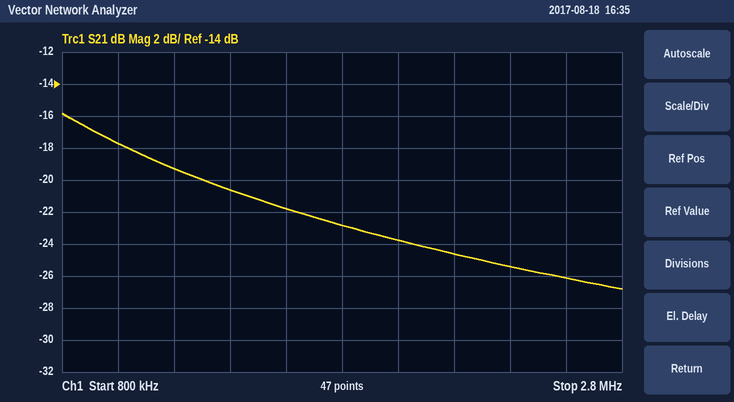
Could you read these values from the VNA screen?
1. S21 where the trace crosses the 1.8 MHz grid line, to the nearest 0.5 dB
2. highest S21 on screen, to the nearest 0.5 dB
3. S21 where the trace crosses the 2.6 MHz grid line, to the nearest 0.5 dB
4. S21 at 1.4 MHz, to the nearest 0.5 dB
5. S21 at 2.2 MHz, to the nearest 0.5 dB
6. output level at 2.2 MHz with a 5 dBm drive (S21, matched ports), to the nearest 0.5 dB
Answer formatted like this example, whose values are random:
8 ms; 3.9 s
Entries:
-23.0 dB; -16.0 dB; -26.0 dB; -20.5 dB; -24.5 dB; -19.5 dBm
